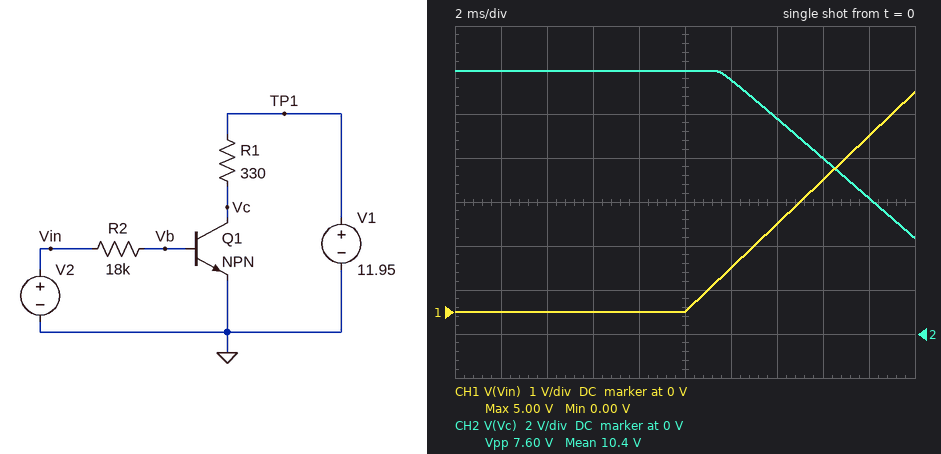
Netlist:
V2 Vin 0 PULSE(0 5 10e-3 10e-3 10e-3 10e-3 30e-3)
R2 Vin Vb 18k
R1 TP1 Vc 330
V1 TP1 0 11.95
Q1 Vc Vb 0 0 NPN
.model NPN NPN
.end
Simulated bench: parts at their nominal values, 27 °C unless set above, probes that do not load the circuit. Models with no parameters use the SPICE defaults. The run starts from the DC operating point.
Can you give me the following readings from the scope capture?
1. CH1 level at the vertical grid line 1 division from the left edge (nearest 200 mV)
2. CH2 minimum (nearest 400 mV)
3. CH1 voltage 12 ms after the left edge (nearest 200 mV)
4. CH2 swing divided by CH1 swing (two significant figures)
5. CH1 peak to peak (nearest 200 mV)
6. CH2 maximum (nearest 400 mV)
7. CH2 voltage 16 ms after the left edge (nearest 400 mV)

0 V
4.4 V
1.0 V
1.5
5.0 V
12.0 V
8.0 V
